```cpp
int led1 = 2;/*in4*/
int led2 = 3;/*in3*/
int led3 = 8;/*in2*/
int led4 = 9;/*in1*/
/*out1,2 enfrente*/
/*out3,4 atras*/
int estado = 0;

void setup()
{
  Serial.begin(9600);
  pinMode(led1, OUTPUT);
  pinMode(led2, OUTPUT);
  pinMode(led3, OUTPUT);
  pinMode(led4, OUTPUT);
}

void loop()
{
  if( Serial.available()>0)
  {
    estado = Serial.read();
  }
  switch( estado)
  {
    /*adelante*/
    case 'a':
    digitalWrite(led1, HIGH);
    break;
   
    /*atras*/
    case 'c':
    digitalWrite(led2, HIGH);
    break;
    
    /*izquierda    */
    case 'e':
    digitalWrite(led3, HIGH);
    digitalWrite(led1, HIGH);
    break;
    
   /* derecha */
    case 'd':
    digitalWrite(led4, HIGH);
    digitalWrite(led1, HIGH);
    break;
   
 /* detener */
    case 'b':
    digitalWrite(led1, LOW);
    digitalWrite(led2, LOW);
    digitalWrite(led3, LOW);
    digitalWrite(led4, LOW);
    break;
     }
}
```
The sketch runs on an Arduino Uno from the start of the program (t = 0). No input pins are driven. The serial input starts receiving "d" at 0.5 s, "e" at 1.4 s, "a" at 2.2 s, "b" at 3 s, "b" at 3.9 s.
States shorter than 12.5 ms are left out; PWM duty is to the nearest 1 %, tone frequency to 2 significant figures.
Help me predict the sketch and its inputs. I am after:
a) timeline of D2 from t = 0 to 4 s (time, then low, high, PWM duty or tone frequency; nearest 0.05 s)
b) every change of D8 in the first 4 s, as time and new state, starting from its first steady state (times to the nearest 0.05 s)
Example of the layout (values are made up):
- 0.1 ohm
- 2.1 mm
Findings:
- 0 s low; 0.5 s high; 3 s low
- 0 s low; 1.4 s high; 3 s low
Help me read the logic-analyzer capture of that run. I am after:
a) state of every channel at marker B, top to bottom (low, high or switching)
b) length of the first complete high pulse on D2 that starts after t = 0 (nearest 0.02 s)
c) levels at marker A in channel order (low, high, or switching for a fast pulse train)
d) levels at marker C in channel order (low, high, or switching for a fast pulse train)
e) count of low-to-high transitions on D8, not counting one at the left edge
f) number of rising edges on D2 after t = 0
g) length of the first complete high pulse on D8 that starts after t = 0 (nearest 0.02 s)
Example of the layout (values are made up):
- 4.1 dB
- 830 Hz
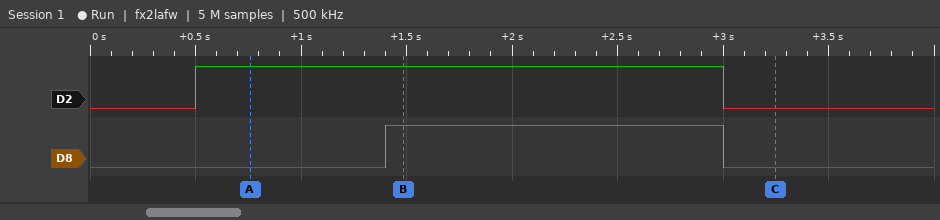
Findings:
- D2 high, D8 high
- 2.50 s
- D2 high, D8 low
- D2 low, D8 low
- 1
- 1
- 1.60 s
